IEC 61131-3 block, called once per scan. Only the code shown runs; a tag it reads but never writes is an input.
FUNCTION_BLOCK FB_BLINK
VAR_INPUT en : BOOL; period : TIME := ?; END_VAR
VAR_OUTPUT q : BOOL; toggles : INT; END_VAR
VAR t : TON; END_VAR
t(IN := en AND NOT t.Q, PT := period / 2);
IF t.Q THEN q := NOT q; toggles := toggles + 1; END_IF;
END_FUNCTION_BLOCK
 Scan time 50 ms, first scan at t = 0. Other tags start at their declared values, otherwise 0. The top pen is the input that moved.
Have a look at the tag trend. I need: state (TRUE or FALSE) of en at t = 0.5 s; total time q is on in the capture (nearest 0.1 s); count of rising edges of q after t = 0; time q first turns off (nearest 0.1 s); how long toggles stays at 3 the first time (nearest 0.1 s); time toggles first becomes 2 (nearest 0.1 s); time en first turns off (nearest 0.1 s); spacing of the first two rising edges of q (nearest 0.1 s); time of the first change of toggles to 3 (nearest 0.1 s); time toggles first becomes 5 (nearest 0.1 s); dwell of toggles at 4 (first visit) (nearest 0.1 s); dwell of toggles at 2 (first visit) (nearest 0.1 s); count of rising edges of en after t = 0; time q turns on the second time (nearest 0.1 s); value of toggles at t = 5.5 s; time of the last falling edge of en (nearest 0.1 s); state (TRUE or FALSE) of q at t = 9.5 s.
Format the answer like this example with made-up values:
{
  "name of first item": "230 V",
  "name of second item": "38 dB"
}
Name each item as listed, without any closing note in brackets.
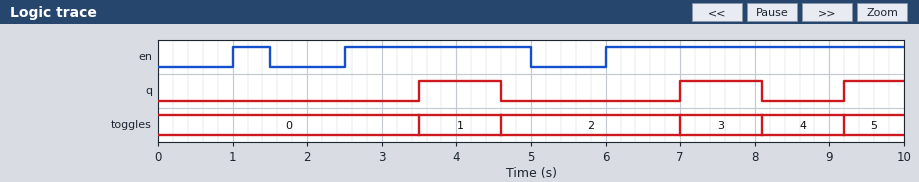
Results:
{
  "state (TRUE or FALSE) of en at t = 0.5 s": "FALSE",
  "total time q is on in the capture": "3.0 s",
  "count of rising edges of q after t = 0": "3",
  "time q first turns off": "4.6 s",
  "how long toggles stays at 3 the first time": "1.1 s",
  "time toggles first becomes 2": "4.6 s",
  "time en first turns off": "1.5 s",
  "spacing of the first two rising edges of q": "3.5 s",
  "time of the first change of toggles to 3": "7.0 s",
  "time toggles first becomes 5": "9.2 s",
  "dwell of toggles at 4 (first visit)": "1.1 s",
  "dwell of toggles at 2 (first visit)": "2.4 s",
  "count of rising edges of en after t = 0": "3",
  "time q turns on the second time": "7.0 s",
  "value of toggles at t = 5.5 s": "2",
  "time of the last falling edge of en": "5.0 s",
  "state (TRUE or FALSE) of q at t = 9.5 s": "TRUE"
}
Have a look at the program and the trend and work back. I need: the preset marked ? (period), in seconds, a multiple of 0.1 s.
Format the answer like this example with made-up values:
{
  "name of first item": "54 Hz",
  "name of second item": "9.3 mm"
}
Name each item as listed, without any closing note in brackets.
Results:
{
  "the preset marked ? (period), in seconds, a multiple of 0.1 s": "2.0 s"
}
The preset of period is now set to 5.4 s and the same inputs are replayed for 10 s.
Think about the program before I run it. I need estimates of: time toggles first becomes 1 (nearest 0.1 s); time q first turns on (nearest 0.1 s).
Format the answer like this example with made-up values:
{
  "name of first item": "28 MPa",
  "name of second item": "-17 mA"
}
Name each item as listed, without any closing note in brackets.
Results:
{
  "time toggles first becomes 1": "8.7 s",
  "time q first turns on": "8.7 s"
}
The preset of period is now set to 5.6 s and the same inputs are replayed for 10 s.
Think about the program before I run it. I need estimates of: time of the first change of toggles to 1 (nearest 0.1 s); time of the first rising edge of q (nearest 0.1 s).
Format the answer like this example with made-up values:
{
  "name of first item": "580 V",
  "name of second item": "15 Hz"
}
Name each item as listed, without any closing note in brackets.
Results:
{
  "time of the first change of toggles to 1": "8.8 s",
  "time of the first rising edge of q": "8.8 s"
}
